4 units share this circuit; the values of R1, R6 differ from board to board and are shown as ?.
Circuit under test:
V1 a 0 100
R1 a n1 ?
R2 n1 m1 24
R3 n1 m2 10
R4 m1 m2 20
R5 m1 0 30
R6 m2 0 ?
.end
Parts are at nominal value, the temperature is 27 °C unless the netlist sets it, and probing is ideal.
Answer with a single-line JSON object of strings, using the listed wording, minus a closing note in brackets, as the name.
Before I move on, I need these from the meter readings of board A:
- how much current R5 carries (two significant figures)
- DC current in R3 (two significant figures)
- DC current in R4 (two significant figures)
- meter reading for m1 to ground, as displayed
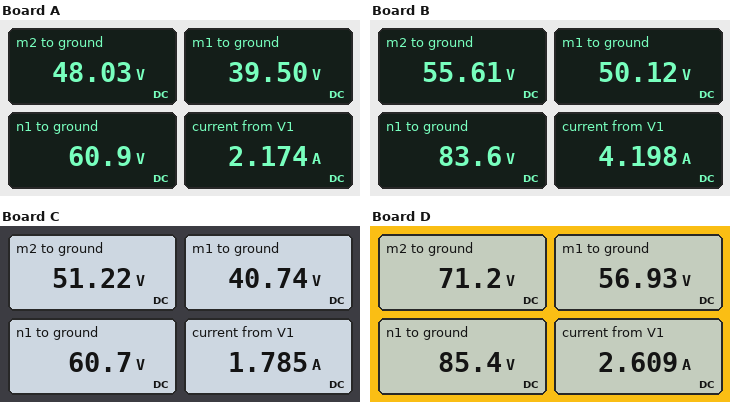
{"how much current R5 carries": "1.3 A", "DC current in R3": "1.3 A", "DC current in R4": "430 mA", "meter reading for m1 to ground, as displayed": "39.50 V"}
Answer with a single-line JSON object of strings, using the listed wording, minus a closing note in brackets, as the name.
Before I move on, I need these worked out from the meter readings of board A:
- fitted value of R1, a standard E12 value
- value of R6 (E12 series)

{"fitted value of R1, a standard E12 value": "18 Ω", "value of R6": "56 Ω"}
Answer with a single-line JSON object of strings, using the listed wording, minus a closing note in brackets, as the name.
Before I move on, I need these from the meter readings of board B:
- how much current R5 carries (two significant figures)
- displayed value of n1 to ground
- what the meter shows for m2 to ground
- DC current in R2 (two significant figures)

{"how much current R5 carries": "1.7 A", "displayed value of n1 to ground": "83.6 V", "what the meter shows for m2 to ground": "55.61 V", "DC current in R2": "1.4 A"}
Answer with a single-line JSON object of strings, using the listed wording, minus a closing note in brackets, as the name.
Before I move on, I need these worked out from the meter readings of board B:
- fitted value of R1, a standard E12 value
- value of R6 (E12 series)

{"fitted value of R1, a standard E12 value": "3.9 Ω", "value of R6": "22 Ω"}
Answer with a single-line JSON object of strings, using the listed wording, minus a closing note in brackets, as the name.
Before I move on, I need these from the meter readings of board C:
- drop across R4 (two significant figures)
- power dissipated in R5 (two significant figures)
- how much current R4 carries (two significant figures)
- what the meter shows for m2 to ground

{"drop across R4": "10 V", "power dissipated in R5": "55 W", "how much current R4 carries": "520 mA", "what the meter shows for m2 to ground": "51.22 V"}
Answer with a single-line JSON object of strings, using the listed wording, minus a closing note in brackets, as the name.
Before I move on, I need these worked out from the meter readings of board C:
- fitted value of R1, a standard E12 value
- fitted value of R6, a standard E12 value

{"fitted value of R1, a standard E12 value": "22 Ω", "fitted value of R6, a standard E12 value": "120 Ω"}
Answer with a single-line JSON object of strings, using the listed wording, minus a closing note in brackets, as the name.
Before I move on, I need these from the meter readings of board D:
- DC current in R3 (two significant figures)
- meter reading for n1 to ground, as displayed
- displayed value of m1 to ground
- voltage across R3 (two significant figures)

{"DC current in R3": "1.4 A", "meter reading for n1 to ground, as displayed": "85.4 V", "displayed value of m1 to ground": "56.93 V", "voltage across R3": "14 V"}
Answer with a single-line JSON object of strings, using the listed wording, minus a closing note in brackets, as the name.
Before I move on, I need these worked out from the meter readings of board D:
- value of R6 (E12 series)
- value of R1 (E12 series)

{"value of R6": "100 Ω", "value of R1": "5.6 Ω"}
